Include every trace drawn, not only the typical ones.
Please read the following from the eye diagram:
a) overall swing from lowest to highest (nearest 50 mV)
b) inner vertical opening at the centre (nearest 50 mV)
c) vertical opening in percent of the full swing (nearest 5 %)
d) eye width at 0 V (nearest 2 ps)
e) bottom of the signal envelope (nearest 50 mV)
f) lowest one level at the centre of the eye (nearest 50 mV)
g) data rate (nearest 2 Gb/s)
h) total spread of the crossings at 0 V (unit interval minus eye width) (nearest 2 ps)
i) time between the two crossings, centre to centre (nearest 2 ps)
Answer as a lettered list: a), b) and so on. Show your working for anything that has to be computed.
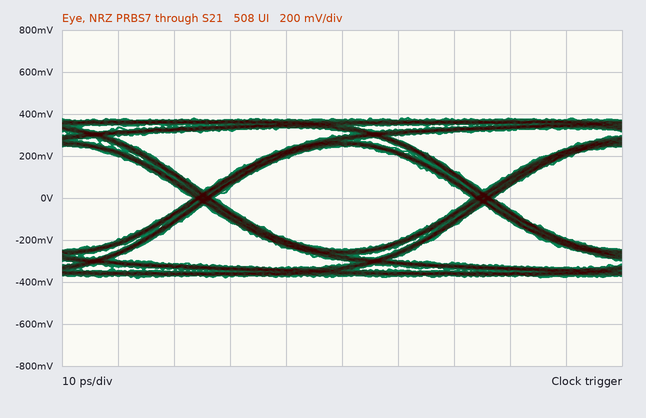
a) 750 mV
b) 500 mV
c) 500 mV / 750 mV ≈ 66.7 %, so 65 % to the nearest 5 %
d) 46 ps
e) -400 mV
f) 250 mV
g) 20 Gb/s
h) 4 ps
i) 50 ps
